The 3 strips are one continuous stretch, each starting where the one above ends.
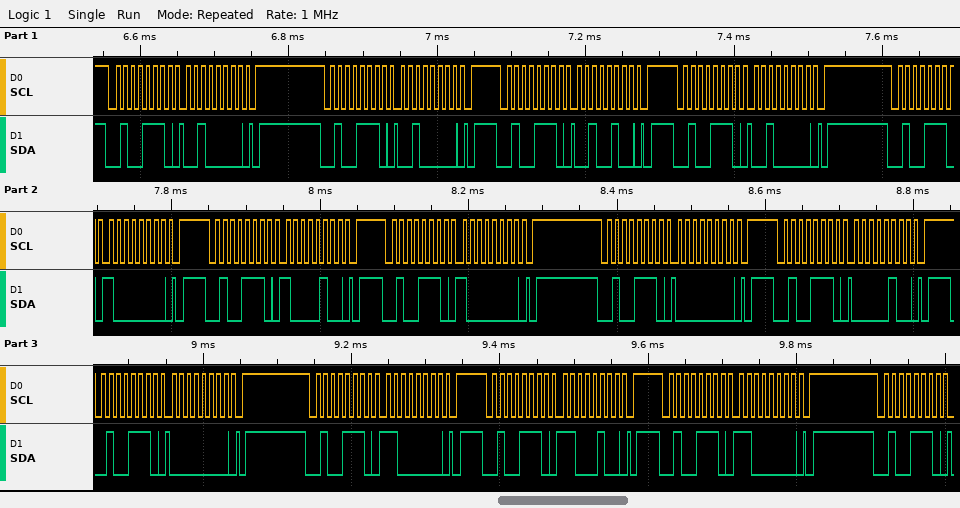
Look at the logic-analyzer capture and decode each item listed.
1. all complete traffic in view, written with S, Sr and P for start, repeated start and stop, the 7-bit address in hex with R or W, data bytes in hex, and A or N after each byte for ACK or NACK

S 27W A 20 A P S 27W A 20 A P S 27W A 24 A P S 27W A 20 A P S 27W A 80 A P S 27W A 84 A P S 27W A 80 A P S 27W A 00 A P S 27W A 04 A P S 27W A 00 A P S 27W A C0 A P S 27W A C4 A P S 27W A C0 A P S 27W A
